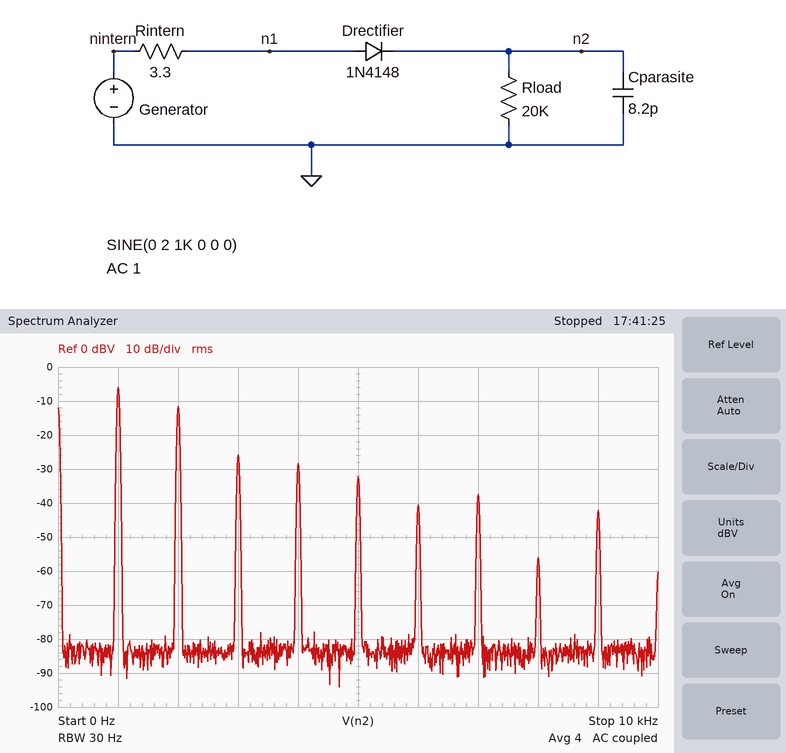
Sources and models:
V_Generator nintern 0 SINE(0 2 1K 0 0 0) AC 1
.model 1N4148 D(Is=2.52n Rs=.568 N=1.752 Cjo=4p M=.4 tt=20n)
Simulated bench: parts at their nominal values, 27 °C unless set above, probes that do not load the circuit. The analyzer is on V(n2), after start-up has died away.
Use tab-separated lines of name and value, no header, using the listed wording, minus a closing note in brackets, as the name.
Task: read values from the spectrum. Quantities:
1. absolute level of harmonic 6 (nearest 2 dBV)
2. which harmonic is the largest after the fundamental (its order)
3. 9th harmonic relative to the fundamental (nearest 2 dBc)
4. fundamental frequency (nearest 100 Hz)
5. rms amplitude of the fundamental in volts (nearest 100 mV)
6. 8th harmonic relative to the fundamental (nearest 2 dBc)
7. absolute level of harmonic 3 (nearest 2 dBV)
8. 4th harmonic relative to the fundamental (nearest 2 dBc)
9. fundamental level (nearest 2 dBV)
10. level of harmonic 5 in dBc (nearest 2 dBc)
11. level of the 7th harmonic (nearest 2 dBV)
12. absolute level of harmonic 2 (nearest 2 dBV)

absolute level of harmonic 6	-40 dBV
which harmonic is the largest after the fundamental	2
9th harmonic relative to the fundamental	-36 dBc
fundamental frequency	1.0 kHz
rms amplitude of the fundamental in volts	500 mV
8th harmonic relative to the fundamental	-50 dBc
absolute level of harmonic 3	-26 dBV
4th harmonic relative to the fundamental	-22 dBc
fundamental level	-6 dBV
level of harmonic 5 in dBc	-26 dBc
level of the 7th harmonic	-38 dBV
absolute level of harmonic 2	-12 dBV
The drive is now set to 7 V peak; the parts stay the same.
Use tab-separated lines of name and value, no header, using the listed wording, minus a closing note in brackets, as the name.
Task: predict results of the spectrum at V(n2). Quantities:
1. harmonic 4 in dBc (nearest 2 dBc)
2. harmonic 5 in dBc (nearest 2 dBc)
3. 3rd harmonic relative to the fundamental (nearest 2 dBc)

harmonic 4 in dBc	-22 dBc
harmonic 5 in dBc	-36 dBc
3rd harmonic relative to the fundamental	-30 dBc
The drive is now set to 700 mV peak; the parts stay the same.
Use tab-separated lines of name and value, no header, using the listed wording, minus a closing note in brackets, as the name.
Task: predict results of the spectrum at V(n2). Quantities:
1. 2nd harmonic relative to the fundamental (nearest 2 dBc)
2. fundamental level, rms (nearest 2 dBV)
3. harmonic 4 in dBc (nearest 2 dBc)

2nd harmonic relative to the fundamental	-4 dBc
fundamental level, rms	-22 dBV
harmonic 4 in dBc	-30 dBc
